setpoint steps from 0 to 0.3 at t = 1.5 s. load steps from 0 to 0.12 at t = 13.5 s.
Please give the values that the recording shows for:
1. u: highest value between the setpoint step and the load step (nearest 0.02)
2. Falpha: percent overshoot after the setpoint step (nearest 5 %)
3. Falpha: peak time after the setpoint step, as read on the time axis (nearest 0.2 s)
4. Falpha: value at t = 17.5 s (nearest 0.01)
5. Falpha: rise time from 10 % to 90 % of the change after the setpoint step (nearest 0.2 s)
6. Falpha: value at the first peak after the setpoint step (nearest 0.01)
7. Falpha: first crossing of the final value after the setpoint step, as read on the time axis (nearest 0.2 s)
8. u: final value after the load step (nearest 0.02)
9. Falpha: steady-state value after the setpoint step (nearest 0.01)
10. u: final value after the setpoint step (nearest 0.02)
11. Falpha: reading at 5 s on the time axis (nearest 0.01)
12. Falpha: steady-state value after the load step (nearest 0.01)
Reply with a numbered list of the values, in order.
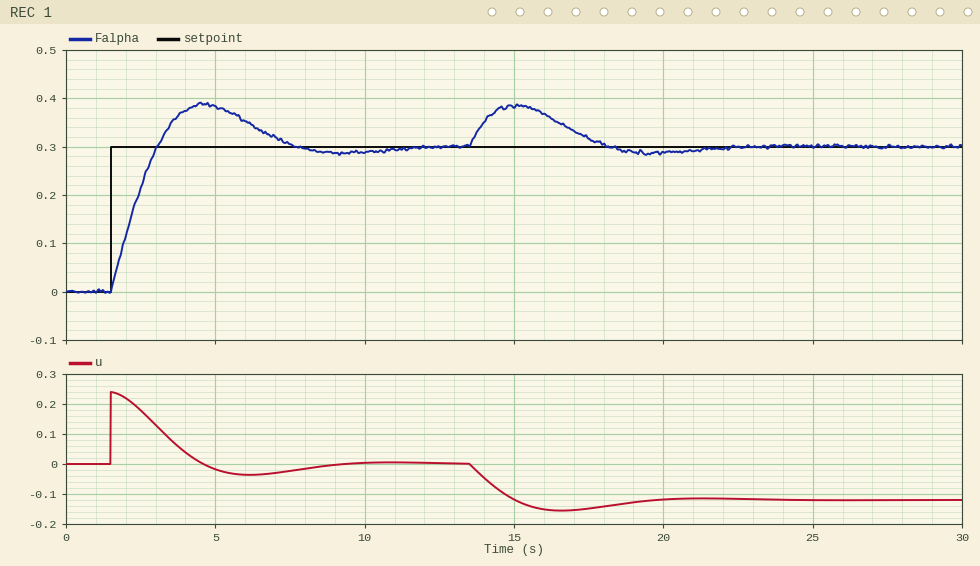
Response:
1. 0.24
2. 30 %
3. 4.6 s
4. 0.32
5. 1.2 s
6. 0.39
7. 3.0 s
8. -0.12
9. 0.30
10. 0.00
11. 0.38
12. 0.30
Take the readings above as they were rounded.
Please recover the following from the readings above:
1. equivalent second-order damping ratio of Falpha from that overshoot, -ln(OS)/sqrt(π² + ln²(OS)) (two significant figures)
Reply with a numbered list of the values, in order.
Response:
1. 0.36
